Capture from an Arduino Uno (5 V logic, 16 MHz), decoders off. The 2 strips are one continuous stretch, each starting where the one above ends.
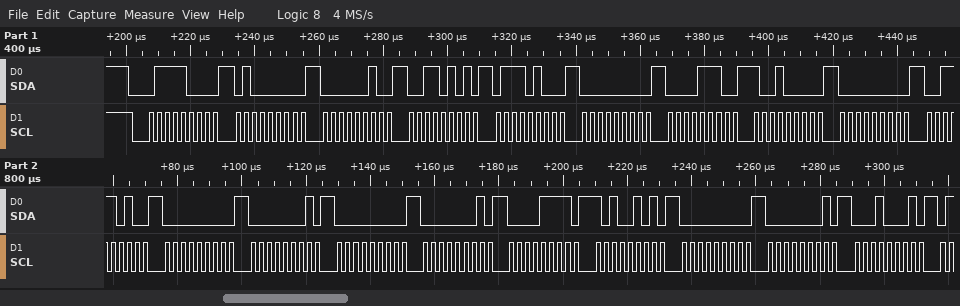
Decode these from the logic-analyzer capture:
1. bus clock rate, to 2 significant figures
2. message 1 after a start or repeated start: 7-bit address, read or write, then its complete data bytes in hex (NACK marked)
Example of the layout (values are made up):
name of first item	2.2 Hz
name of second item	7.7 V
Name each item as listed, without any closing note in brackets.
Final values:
bus clock rate, to 2 significant figures	400 kHz
message 1 after a start or repeated start: 7-bit address, read or write, then its complete data bytes in hex	0x3C write: 40 02 35 74 00 0E 90 00 3A 00 01 00 01 0F A5 00 01 11
